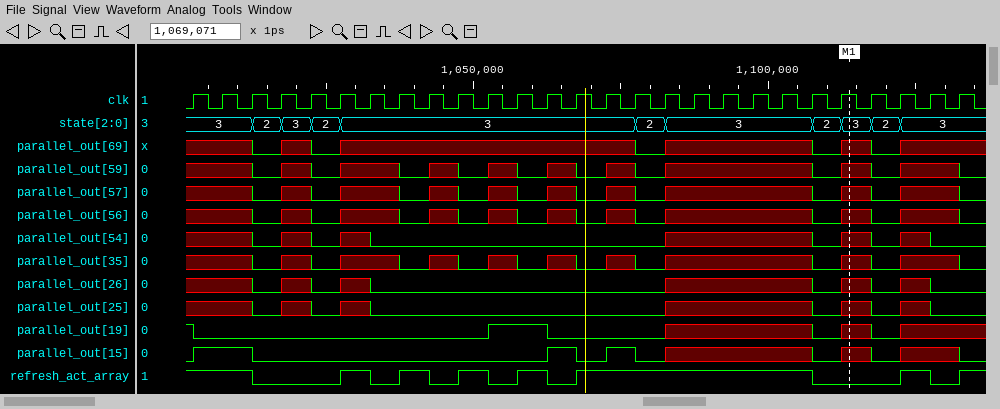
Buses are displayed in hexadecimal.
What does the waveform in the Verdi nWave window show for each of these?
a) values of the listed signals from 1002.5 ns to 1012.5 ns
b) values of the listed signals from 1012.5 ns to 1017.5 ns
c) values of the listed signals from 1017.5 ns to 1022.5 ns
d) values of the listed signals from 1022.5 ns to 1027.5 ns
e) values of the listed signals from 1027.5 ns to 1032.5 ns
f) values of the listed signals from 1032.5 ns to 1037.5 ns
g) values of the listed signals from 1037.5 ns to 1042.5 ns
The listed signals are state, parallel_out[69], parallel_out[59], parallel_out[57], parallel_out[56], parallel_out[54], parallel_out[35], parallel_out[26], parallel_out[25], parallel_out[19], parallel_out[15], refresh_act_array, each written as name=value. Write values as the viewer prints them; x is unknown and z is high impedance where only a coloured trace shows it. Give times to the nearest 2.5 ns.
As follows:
state=3, parallel_out[69]=x, parallel_out[59]=x, parallel_out[57]=x, parallel_out[56]=x, parallel_out[54]=x, parallel_out[35]=x, parallel_out[26]=x, parallel_out[25]=x, parallel_out[19]=0, parallel_out[15]=1, refresh_act_array=1
state=2, parallel_out[69]=0, parallel_out[59]=0, parallel_out[57]=0, parallel_out[56]=0, parallel_out[54]=0, parallel_out[35]=0, parallel_out[26]=0, parallel_out[25]=0, parallel_out[19]=0, parallel_out[15]=0, refresh_act_array=0
state=3, parallel_out[69]=x, parallel_out[59]=x, parallel_out[57]=x, parallel_out[56]=x, parallel_out[54]=x, parallel_out[35]=x, parallel_out[26]=x, parallel_out[25]=x, parallel_out[19]=0, parallel_out[15]=0, refresh_act_array=0
state=2, parallel_out[69]=0, parallel_out[59]=0, parallel_out[57]=0, parallel_out[56]=0, parallel_out[54]=0, parallel_out[35]=0, parallel_out[26]=0, parallel_out[25]=0, parallel_out[19]=0, parallel_out[15]=0, refresh_act_array=0
state=3, parallel_out[69]=x, parallel_out[59]=x, parallel_out[57]=x, parallel_out[56]=x, parallel_out[54]=x, parallel_out[35]=x, parallel_out[26]=x, parallel_out[25]=x, parallel_out[19]=0, parallel_out[15]=0, refresh_act_array=1
state=3, parallel_out[69]=x, parallel_out[59]=x, parallel_out[57]=x, parallel_out[56]=x, parallel_out[54]=0, parallel_out[35]=x, parallel_out[26]=0, parallel_out[25]=0, parallel_out[19]=0, parallel_out[15]=0, refresh_act_array=0
state=3, parallel_out[69]=x, parallel_out[59]=0, parallel_out[57]=0, parallel_out[56]=0, parallel_out[54]=0, parallel_out[35]=0, parallel_out[26]=0, parallel_out[25]=0, parallel_out[19]=0, parallel_out[15]=0, refresh_act_array=1
